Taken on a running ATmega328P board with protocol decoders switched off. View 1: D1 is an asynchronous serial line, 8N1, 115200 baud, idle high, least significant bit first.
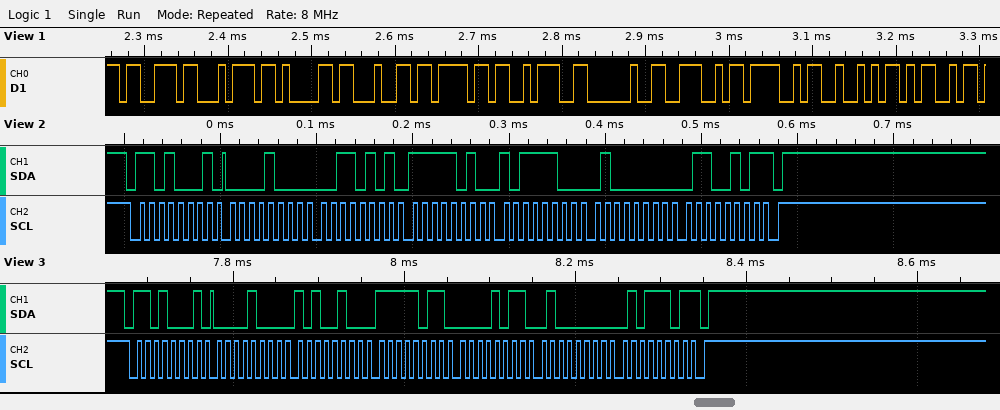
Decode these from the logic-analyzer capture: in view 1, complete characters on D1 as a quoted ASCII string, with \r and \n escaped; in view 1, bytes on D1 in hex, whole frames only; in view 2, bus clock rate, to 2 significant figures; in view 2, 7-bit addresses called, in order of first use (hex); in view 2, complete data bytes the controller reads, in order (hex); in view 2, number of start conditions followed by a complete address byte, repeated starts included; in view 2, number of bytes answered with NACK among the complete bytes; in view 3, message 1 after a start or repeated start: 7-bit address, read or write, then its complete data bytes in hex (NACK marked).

"stado: NORM"
73 74 61 64 6F 3A 20 4E 4F 52 4D
100 kHz
0x68
08 35 FA BC 40 65
1
1
0x68 read: 08 A4 FB 0B 40 5D NACK
